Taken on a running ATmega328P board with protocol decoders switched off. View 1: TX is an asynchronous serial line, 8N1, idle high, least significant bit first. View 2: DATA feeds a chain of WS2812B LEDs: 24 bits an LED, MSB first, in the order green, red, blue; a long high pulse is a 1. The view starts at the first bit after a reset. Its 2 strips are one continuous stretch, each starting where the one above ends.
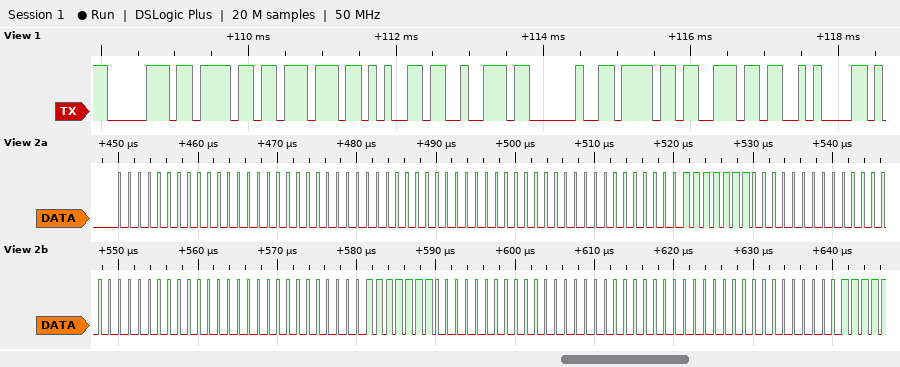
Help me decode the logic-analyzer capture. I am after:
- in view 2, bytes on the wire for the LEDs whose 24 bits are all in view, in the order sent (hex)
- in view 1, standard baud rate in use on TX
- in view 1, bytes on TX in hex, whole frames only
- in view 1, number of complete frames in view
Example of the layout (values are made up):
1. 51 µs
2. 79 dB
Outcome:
1. 00 00 00 00 00 00 00 7F 00 00 00 00 00 7F 00 00 00 00
2. 9600 baud
3. 70 6F 77 65 72 20 6F 6E 0A
4. 9
